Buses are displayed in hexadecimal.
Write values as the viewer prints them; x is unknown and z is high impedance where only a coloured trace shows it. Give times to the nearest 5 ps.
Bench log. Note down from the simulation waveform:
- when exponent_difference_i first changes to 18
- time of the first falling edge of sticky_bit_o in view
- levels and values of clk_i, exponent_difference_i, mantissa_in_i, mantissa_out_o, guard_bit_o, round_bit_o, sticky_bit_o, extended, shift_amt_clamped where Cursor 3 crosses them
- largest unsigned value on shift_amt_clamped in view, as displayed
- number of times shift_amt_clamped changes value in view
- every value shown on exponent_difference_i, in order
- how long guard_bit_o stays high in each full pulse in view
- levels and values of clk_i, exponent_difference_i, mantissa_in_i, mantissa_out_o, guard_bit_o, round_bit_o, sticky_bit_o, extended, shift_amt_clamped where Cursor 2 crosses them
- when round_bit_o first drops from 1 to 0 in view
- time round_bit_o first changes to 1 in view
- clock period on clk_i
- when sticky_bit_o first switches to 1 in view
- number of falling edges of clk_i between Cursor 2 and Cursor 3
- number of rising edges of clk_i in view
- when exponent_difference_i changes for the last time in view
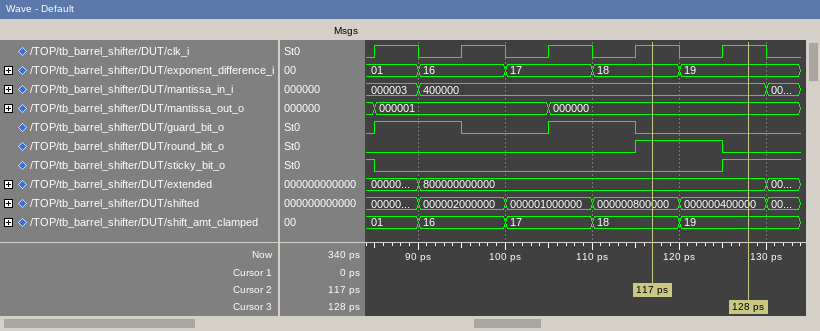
110 ps
85 ps
clk_i=1, exponent_difference_i=19, mantissa_in_i=400000, mantissa_out_o=000000, guard_bit_o=0, round_bit_o=0, sticky_bit_o=1, extended=800000000000, shift_amt_clamped=19
19
4
01, 16, 17, 18, 19
10 ps, 10 ps
clk_i=1, exponent_difference_i=18, mantissa_in_i=400000, mantissa_out_o=000000, guard_bit_o=0, round_bit_o=1, sticky_bit_o=0, extended=800000000000, shift_amt_clamped=18
125 ps
115 ps
10 ps
125 ps
1
5
120 ps
